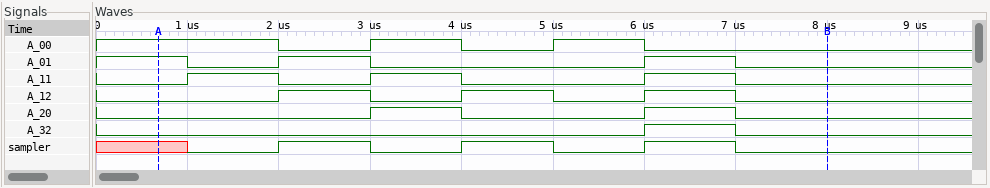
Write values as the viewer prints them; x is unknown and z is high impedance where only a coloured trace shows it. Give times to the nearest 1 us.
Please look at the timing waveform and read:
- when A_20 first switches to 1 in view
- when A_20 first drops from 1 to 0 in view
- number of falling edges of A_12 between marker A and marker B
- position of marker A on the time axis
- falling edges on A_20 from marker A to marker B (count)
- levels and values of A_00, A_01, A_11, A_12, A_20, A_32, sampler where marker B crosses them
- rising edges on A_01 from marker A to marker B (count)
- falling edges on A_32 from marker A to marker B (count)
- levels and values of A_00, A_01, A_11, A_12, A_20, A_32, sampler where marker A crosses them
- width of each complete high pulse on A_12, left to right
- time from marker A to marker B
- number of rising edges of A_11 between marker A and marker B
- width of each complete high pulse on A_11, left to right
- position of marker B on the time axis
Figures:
3 us
4 us
3
1 us
2
A_00=0, A_01=0, A_11=0, A_12=0, A_20=0, A_32=0, sampler=0
2
1
A_00=1, A_01=1, A_11=0, A_12=0, A_20=0, A_32=0, sampler=x
1 us, 1 us, 1 us
7 us
3
1 us, 1 us, 1 us
8 us
